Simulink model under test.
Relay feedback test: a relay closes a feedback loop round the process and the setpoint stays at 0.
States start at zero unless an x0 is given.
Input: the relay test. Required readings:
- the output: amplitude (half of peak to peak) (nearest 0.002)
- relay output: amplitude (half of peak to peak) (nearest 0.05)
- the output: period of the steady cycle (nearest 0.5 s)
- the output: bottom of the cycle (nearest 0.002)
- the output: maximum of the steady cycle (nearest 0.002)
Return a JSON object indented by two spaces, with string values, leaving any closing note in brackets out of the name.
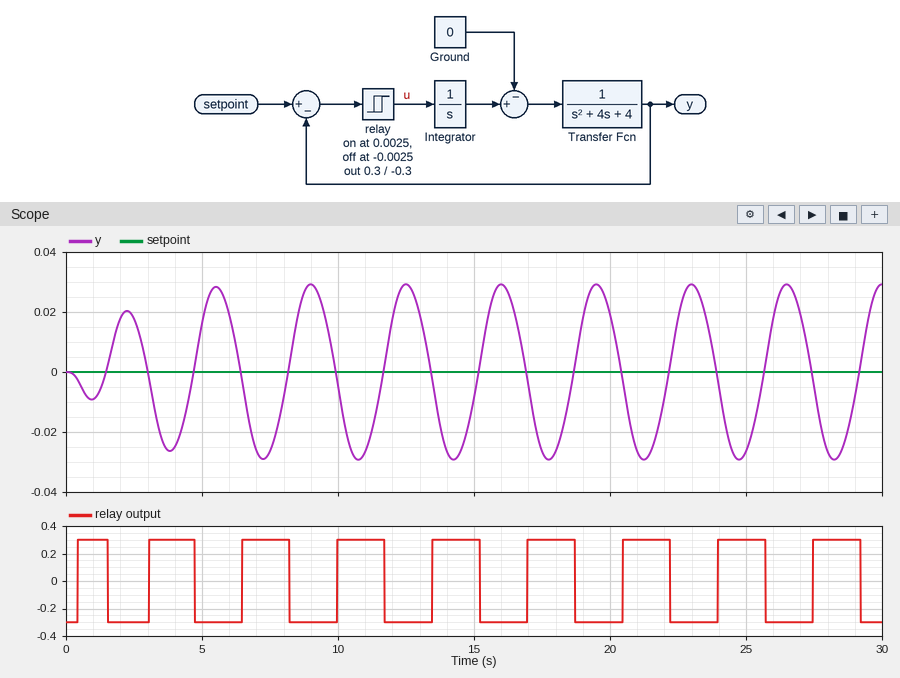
{
  "the output: amplitude (half of peak to peak)": "0.030",
  "relay output: amplitude (half of peak to peak)": "0.30",
  "the output: period of the steady cycle": "3.5 s",
  "the output: bottom of the cycle": "-0.030",
  "the output: maximum of the steady cycle": "0.030"
}
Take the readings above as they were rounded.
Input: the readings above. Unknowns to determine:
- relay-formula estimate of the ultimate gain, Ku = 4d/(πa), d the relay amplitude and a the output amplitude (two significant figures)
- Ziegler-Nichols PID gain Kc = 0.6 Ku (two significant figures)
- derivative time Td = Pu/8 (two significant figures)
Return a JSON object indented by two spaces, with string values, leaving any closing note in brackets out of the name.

{
  "relay-formula estimate of the ultimate gain, Ku = 4d/(πa), d the relay amplitude and a the output amplitude": "13",
  "Ziegler-Nichols PID gain Kc = 0.6 Ku": "7.8",
  "derivative time Td = Pu/8": "0.44 s"
}
